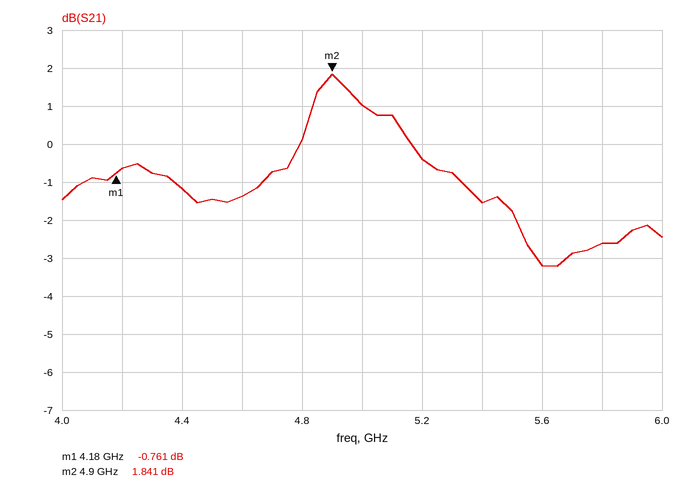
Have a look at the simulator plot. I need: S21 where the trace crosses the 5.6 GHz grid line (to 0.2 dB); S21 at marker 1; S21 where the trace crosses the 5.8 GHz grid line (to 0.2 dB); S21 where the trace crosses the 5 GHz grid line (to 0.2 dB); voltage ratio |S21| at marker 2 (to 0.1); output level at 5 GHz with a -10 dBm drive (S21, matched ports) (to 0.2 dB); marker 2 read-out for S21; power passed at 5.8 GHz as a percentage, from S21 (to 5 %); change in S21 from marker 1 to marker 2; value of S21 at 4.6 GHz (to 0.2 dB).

-3.2 dB
-0.761 dB
-2.6 dB
1.0 dB
1.2
-9.0 dBm
1.841 dB
55 %
2.602 dB
-1.4 dB
